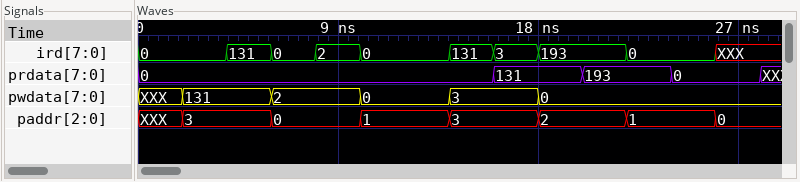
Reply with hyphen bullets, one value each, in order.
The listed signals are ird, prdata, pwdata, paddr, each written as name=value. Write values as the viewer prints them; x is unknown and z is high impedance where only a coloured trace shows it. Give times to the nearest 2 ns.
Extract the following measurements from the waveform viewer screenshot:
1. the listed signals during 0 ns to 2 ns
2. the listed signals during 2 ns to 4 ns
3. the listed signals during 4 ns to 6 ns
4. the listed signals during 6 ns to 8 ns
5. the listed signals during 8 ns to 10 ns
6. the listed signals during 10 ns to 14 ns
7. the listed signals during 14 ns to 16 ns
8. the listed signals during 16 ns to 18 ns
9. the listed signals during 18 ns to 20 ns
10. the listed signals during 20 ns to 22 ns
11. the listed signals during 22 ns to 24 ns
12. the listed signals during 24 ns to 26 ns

- ird=0, prdata=0, pwdata=XXX, paddr=XXX
- ird=0, prdata=0, pwdata=131, paddr=3
- ird=131, prdata=0, pwdata=131, paddr=3
- ird=0, prdata=0, pwdata=2, paddr=0
- ird=2, prdata=0, pwdata=2, paddr=0
- ird=0, prdata=0, pwdata=0, paddr=1
- ird=131, prdata=0, pwdata=3, paddr=3
- ird=3, prdata=131, pwdata=3, paddr=3
- ird=193, prdata=131, pwdata=0, paddr=2
- ird=193, prdata=193, pwdata=0, paddr=2
- ird=0, prdata=193, pwdata=0, paddr=1
- ird=0, prdata=0, pwdata=0, paddr=1
